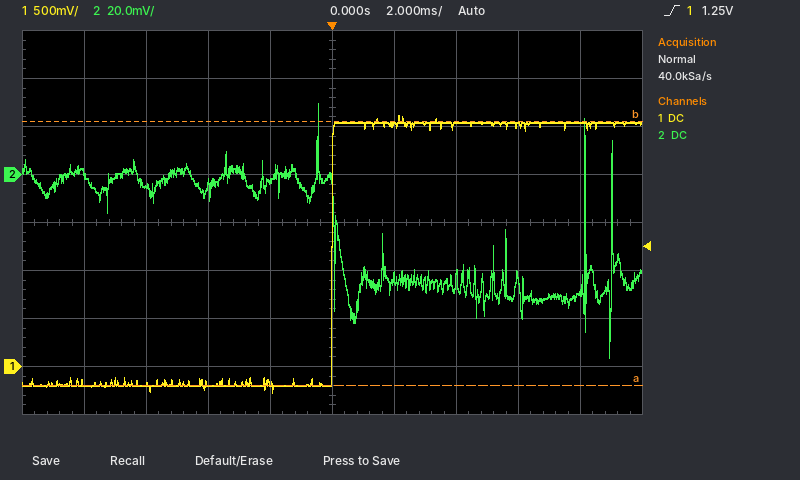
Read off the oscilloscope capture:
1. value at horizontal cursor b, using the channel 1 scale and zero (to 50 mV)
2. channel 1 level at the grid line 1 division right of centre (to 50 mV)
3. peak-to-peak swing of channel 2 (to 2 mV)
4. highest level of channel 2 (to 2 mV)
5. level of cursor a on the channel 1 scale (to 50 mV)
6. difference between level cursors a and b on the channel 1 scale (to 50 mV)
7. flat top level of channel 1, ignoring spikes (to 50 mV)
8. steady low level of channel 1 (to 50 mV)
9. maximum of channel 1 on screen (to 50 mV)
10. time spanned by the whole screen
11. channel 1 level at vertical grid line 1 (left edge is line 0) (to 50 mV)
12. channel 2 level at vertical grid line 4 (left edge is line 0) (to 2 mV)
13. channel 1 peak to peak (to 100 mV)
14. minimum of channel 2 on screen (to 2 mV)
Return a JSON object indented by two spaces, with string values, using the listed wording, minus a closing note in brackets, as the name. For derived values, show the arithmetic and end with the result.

{
  "value at horizontal cursor b, using the channel 1 scale and zero": "2.55 V",
  "channel 1 level at the grid line 1 division right of centre": "2.50 V",
  "peak-to-peak swing of channel 2": "30 mV − (-76 mV) = 106 mV",
  "highest level of channel 2": "30 mV",
  "level of cursor a on the channel 1 scale": "-200 mV",
  "difference between level cursors a and b on the channel 1 scale": "2.75 V",
  "flat top level of channel 1, ignoring spikes": "2.55 V",
  "steady low level of channel 1": "-200 mV",
  "maximum of channel 1 on screen": "2.60 V",
  "time spanned by the whole screen": "20 ms",
  "channel 1 level at vertical grid line 1 (left edge is line 0)": "-150 mV",
  "channel 2 level at vertical grid line 4 (left edge is line 0)": "-2 mV",
  "channel 1 peak to peak": "2.90 V",
  "minimum of channel 2 on screen": "-76 mV"
}
